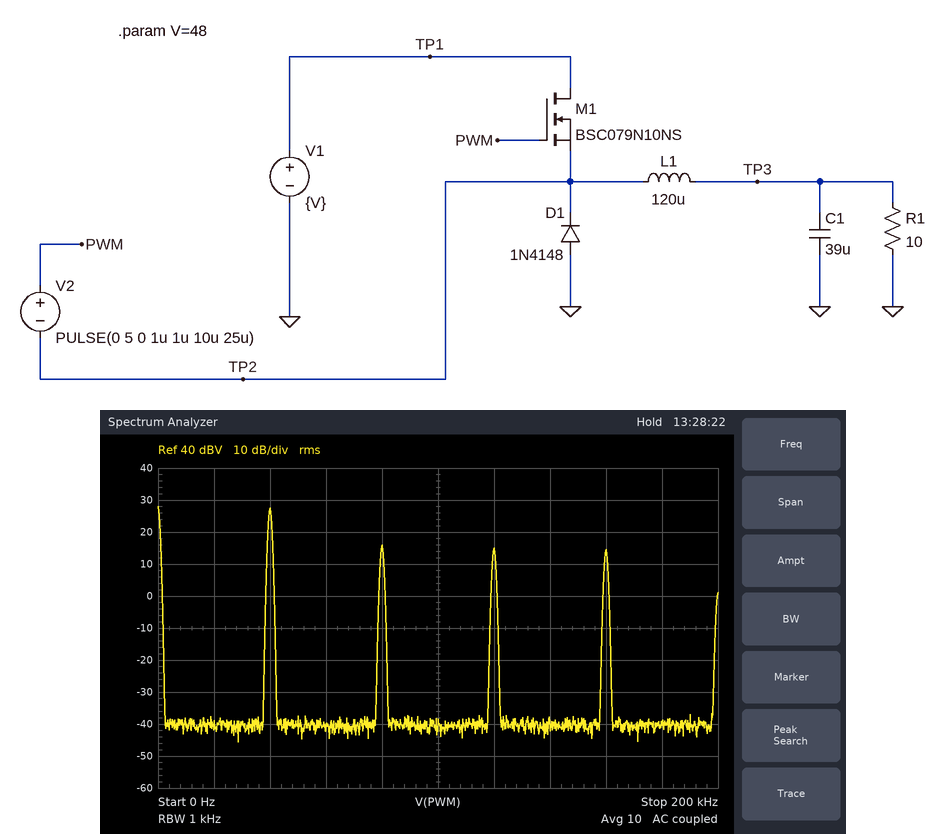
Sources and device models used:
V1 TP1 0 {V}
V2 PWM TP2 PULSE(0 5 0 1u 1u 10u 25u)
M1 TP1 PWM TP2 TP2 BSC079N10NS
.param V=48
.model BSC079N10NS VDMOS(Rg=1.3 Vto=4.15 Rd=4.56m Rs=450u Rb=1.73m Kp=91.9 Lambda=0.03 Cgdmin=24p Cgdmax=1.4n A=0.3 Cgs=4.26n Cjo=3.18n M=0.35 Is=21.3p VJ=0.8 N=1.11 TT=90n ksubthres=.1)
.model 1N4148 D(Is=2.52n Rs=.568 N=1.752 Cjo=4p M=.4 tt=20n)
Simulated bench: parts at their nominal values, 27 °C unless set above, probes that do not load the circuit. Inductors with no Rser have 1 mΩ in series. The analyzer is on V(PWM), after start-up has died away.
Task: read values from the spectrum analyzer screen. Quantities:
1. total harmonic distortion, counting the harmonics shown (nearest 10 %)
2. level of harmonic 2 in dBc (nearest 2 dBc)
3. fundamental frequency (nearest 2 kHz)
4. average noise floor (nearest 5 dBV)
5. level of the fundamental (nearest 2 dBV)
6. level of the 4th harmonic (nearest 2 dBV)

40 %
-12 dBc
40 kHz
-40 dBV
28 dBV
14 dBV
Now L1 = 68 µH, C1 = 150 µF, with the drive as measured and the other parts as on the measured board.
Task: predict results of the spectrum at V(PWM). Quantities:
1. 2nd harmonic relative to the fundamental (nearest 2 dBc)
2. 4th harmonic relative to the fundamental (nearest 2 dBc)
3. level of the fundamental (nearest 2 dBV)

-14 dBc
-16 dBc
28 dBV
